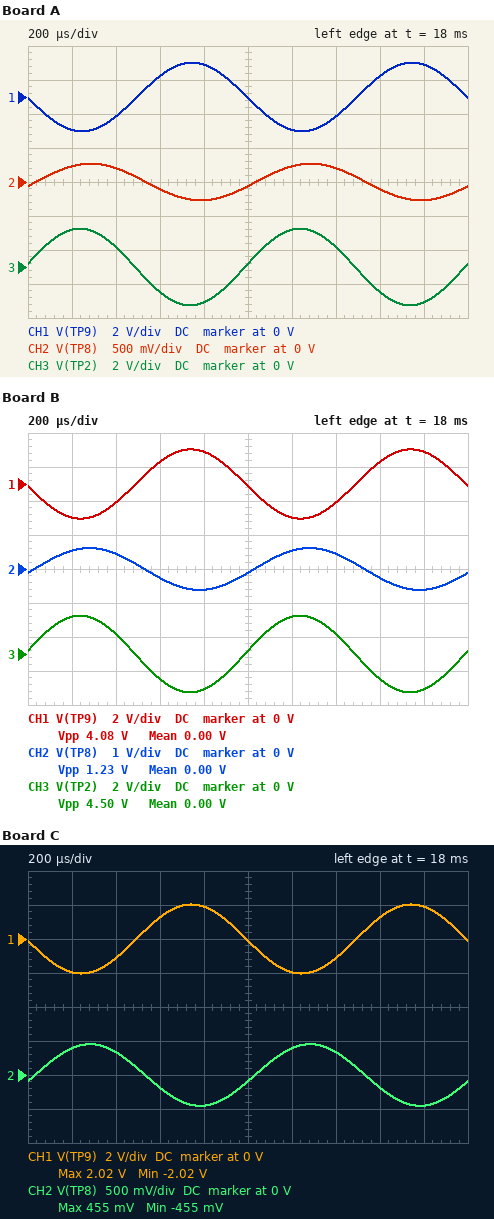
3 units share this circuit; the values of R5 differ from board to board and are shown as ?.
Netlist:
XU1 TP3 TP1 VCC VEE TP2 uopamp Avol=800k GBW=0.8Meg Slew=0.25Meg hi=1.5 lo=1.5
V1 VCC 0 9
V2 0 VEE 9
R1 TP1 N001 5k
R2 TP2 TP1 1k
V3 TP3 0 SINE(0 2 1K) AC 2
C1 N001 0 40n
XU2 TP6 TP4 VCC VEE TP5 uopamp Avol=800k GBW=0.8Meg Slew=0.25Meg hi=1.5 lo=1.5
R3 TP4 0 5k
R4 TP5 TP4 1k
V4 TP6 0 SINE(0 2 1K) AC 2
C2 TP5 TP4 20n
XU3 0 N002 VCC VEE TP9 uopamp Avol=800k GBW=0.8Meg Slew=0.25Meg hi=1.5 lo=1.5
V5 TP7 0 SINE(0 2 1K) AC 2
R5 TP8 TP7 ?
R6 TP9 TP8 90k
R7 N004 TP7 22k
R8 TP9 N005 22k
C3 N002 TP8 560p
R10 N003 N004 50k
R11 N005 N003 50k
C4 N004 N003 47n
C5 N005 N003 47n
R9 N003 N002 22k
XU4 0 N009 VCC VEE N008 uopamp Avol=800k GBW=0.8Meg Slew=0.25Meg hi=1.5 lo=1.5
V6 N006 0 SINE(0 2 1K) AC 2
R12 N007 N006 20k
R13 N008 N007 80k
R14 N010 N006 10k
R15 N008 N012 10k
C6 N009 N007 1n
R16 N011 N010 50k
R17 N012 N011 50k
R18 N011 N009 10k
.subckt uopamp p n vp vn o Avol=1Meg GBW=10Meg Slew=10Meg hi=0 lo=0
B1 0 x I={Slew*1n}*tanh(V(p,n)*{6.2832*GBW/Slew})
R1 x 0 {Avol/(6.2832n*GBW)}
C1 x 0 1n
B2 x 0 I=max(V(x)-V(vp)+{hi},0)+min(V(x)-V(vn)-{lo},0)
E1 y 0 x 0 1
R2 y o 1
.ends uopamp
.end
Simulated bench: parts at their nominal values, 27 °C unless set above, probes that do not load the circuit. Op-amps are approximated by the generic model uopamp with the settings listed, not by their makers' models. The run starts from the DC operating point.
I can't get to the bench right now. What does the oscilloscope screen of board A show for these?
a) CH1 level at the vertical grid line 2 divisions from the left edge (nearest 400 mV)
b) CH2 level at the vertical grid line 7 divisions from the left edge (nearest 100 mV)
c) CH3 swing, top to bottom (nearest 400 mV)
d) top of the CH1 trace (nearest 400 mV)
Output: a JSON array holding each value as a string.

["-1.2 V", "200 mV", "4.4 V", "2.0 V"]
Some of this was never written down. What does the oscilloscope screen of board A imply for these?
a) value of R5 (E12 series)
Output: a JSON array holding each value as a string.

["68 kΩ"]
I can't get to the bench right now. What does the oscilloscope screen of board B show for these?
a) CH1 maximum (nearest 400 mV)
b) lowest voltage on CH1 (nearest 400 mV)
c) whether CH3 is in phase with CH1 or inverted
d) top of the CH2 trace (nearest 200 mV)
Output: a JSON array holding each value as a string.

["2.0 V", "-2.0 V", "inverted", "600 mV"]
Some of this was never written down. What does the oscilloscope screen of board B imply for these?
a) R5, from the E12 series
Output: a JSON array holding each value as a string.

["47 kΩ"]
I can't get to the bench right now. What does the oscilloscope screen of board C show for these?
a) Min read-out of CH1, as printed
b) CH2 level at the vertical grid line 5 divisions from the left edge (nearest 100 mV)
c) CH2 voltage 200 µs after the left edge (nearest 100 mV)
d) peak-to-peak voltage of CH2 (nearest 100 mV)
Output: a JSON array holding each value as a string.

["-2.02 V", "-100 mV", "400 mV", "900 mV"]
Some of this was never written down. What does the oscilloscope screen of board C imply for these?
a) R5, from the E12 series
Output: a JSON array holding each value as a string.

["56 kΩ"]
